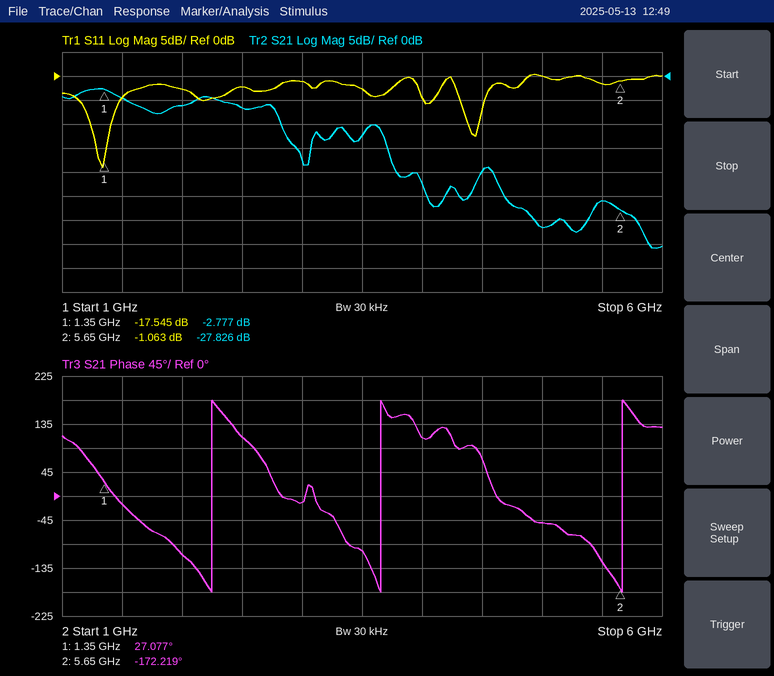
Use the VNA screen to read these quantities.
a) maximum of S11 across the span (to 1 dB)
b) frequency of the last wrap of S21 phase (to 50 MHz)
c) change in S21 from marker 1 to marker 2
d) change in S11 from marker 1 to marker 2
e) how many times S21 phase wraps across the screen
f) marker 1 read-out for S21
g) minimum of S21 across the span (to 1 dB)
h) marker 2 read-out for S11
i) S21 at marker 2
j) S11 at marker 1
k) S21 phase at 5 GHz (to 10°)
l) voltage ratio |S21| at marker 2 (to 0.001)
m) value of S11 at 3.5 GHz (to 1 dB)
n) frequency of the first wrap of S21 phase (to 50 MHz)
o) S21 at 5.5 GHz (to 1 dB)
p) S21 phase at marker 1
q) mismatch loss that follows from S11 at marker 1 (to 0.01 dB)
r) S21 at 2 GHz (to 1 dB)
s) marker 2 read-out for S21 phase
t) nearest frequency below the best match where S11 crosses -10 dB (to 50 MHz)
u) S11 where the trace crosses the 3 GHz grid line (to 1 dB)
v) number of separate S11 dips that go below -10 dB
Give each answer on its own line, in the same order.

0 dB
5.65 GHz
-25.049 dB
16.482 dB
3
-2.777 dB
-36 dB
-1.063 dB
-27.826 dB
-17.545 dB
-50°
0.041
-3 dB
2.25 GHz
-26 dB
27.077°
0.08 dB
-6 dB
-172.219°
1.25 GHz
-1 dB
2
